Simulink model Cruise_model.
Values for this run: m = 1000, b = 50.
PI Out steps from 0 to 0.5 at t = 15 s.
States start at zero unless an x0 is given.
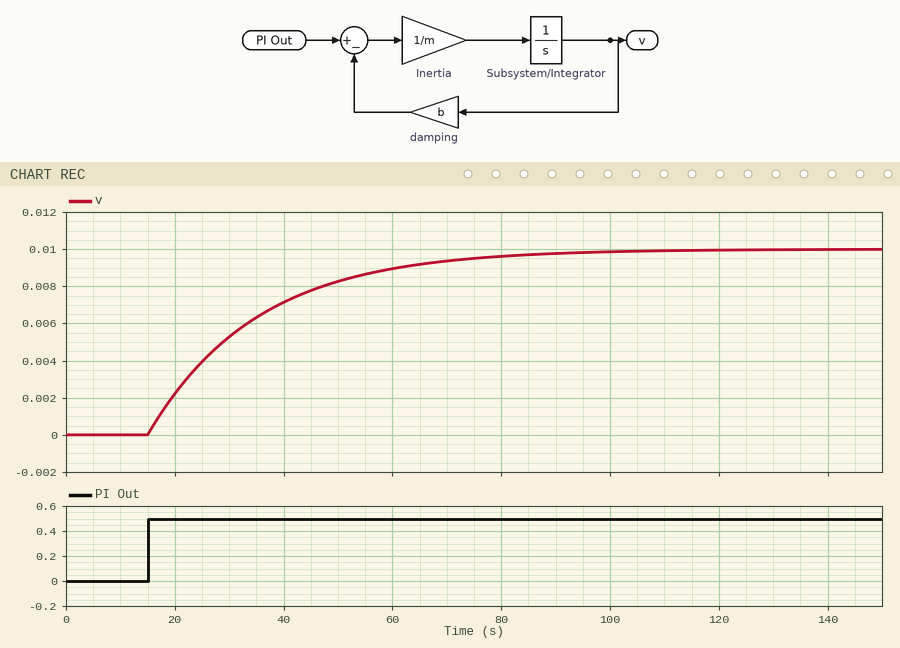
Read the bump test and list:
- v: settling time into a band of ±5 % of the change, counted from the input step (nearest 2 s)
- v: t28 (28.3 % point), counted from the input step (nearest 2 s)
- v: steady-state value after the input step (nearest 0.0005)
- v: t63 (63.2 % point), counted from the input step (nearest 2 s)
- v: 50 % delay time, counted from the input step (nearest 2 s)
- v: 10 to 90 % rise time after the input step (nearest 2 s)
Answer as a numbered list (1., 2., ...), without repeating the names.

1. 60 s
2. 6 s
3. 0.0100
4. 20 s
5. 14 s
6. 44 s
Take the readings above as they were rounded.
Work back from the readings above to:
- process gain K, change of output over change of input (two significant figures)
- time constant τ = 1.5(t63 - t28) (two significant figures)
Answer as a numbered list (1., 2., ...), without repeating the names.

1. 0.020
2. 21 s
